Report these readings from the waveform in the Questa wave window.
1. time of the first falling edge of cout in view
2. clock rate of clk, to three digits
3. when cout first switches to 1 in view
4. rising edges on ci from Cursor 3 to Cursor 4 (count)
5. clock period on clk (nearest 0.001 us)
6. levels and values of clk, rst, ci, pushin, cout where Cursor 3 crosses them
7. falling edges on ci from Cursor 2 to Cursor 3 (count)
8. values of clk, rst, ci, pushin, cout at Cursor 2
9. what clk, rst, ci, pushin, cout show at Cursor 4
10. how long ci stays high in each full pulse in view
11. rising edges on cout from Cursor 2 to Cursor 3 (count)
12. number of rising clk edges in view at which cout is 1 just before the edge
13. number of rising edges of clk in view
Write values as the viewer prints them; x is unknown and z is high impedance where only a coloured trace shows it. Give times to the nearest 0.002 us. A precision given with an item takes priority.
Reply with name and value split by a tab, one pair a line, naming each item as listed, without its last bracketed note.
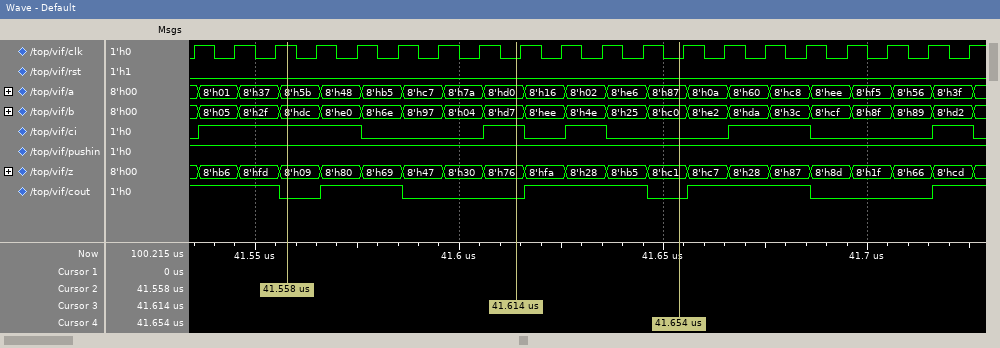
time of the first falling edge of cout in view	41.556 us
clock rate of clk, to three digits	100 MHz
when cout first switches to 1 in view	41.566 us
rising edges on ci from Cursor 3 to Cursor 4	1
clock period on clk	0.01 us
levels and values of clk, rst, ci, pushin, cout where Cursor 3 crosses them	clk=0, rst=0, ci=1, pushin=1, cout=0
falling edges on ci from Cursor 2 to Cursor 3	1
values of clk, rst, ci, pushin, cout at Cursor 2	clk=1, rst=0, ci=1, pushin=1, cout=0
what clk, rst, ci, pushin, cout show at Cursor 4	clk=0, rst=0, ci=0, pushin=1, cout=0
how long ci stays high in each full pulse in view	0.04 us, 0.01 us, 0.01 us, 0.02 us, 0.01 us
rising edges on cout from Cursor 2 to Cursor 3	1
number of rising clk edges in view at which cout is 1 just before the edge	12
number of rising edges of clk in view	20
